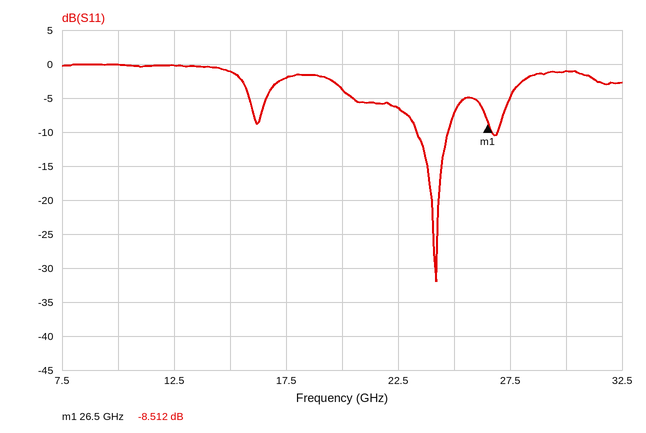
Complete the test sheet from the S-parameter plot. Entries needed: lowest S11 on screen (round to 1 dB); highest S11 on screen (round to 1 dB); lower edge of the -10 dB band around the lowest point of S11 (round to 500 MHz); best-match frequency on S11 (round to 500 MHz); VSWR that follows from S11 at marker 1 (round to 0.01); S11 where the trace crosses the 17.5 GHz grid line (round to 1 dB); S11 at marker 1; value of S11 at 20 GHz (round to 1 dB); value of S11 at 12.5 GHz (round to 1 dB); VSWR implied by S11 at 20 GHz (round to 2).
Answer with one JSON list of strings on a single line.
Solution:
["-32 dB", "0 dB", "23.5 GHz", "24.0 GHz", "2.20", "-2 dB", "-8.512 dB", "-4 dB", "0 dB", "4"]
